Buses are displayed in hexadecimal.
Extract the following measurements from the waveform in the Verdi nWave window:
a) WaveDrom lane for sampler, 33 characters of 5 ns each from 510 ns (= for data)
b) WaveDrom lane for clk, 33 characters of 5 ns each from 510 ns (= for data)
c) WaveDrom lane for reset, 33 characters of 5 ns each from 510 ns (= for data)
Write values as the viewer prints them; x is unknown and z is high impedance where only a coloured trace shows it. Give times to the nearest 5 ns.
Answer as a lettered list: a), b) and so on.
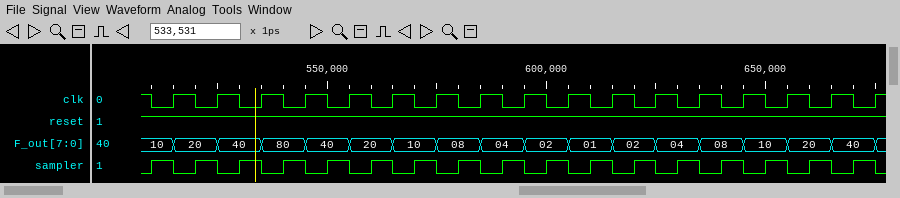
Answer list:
a) {name: 'sampler', wave: '101010101010101010101010101010101'}
b) {name: 'clk', wave: '010101010101010101010101010101010'}
c) {name: 'reset', wave: '1................................'}
